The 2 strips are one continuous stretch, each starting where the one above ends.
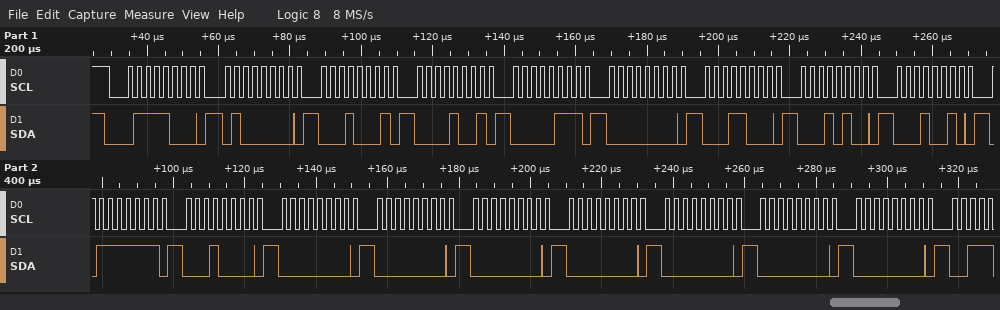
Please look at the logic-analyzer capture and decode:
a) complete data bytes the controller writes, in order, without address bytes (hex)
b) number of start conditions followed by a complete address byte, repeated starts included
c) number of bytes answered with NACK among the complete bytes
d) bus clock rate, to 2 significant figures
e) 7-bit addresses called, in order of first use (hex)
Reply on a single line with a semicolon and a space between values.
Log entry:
40 11 09 07 00 18 14 12 7F 10 00 00 00 00 00 00 00; 1; 0; 400 kHz; 0x3C
